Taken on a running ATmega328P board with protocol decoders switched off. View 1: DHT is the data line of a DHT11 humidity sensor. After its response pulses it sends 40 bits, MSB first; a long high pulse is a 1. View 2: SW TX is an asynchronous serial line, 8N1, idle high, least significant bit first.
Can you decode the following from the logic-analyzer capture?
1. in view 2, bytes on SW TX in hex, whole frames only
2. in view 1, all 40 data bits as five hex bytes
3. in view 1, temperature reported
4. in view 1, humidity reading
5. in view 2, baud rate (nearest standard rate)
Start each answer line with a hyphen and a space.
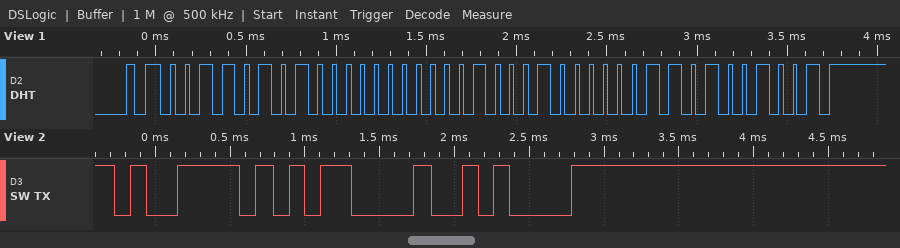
- 79 0D 0A
- 35 00 11 03 49
- 17.3 °C
- 53 %
- 9600 baud
